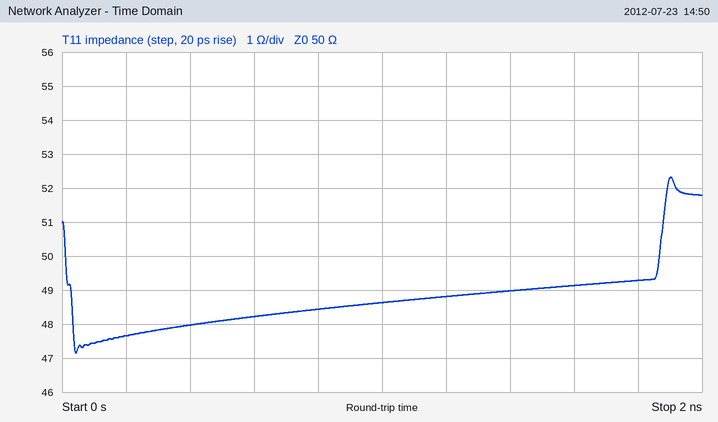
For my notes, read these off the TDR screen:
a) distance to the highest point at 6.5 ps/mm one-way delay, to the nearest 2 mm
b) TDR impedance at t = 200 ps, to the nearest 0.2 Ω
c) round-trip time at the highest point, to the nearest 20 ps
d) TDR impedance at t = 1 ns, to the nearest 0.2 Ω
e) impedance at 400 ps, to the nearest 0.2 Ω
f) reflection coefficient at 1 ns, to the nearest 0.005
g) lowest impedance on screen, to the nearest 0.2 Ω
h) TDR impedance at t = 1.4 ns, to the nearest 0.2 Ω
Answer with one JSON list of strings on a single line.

["146 mm", "47.6 Ω", "1.90 ns", "48.6 Ω", "48.0 Ω", "-0.015", "47.2 Ω", "49.0 Ω"]
